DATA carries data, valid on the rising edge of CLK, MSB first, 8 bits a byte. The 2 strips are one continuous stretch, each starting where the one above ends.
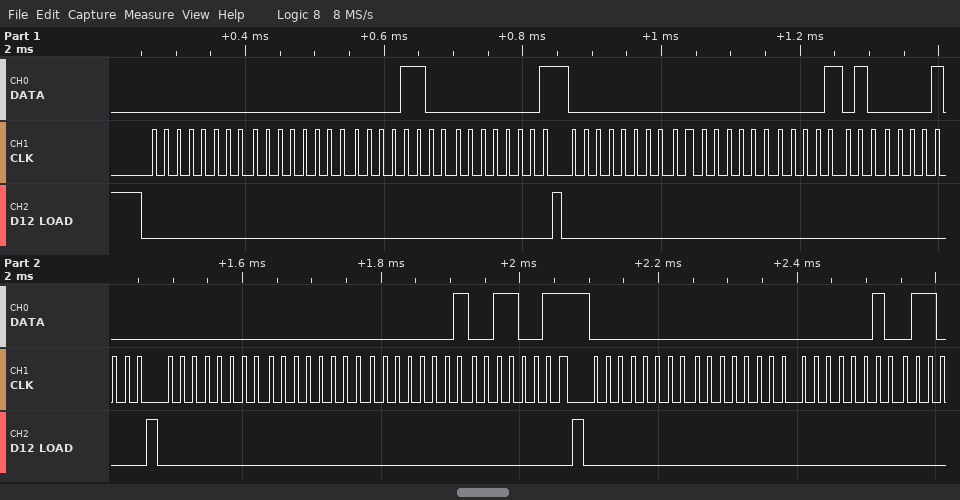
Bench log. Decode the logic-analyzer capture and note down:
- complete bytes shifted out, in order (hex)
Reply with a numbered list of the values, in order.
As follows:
1. 0x00 0x00 0x0C 0x01 0x00 0x00 0x0A 0x08 0x00 0x00 0x01 0x33 0x00 0x00 0x02
